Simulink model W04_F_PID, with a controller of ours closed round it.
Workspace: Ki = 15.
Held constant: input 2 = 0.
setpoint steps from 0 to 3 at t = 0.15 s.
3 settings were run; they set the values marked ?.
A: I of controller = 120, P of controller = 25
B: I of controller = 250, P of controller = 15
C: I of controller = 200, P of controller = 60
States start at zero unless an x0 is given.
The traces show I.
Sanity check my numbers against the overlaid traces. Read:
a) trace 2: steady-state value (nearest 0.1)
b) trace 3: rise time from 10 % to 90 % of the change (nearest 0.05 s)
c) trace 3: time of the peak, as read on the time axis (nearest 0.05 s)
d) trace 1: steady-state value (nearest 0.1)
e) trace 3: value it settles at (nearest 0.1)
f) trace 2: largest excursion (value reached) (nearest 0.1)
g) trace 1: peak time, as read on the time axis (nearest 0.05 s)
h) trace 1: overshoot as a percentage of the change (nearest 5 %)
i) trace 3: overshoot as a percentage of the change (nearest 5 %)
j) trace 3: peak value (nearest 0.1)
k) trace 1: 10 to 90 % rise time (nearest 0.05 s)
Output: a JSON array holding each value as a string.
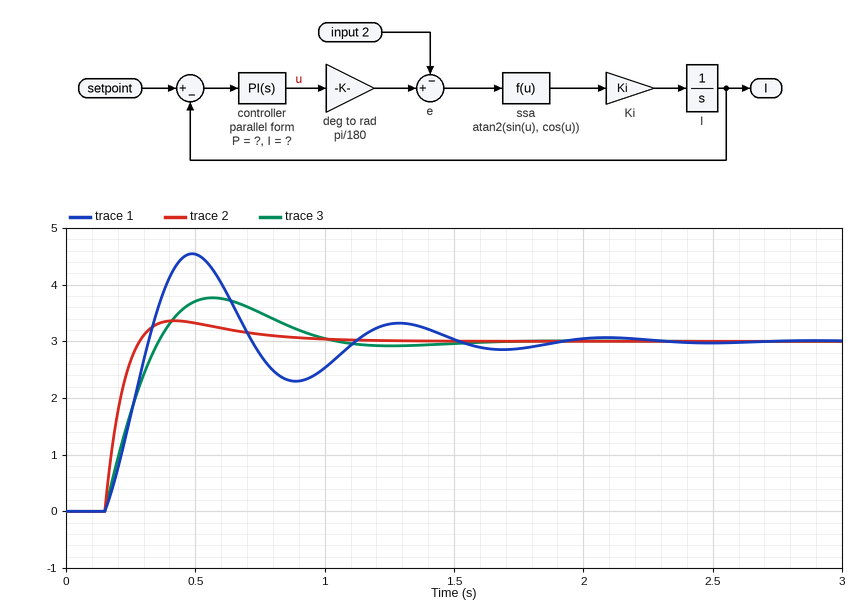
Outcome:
["3.0", "0.15 s", "0.55 s", "3.0", "3.0", "3.4", "0.50 s", "50 %", "25 %", "3.8", "0.15 s"]
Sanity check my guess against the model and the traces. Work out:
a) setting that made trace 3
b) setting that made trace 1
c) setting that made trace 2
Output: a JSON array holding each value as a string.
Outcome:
["A", "B", "C"]
